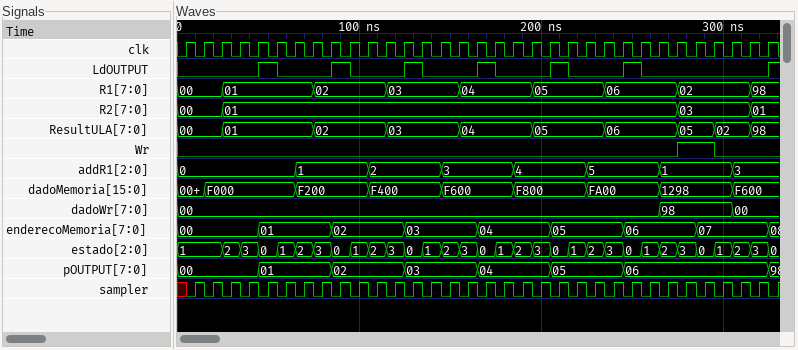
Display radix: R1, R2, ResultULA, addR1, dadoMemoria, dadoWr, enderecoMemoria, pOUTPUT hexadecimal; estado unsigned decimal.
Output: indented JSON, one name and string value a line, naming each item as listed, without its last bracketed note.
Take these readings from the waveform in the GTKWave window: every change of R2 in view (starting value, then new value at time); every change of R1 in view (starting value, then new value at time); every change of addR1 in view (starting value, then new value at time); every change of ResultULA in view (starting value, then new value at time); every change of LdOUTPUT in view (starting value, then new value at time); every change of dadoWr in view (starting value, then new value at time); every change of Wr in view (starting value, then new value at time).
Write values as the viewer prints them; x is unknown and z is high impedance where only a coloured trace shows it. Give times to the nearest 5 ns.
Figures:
{
  "every change of R2 in view": "00, 01 at 25 ns, 03 at 275 ns, 01 at 315 ns",
  "every change of R1 in view": "00, 01 at 25 ns, 02 at 75 ns, 03 at 115 ns, 04 at 155 ns, 05 at 195 ns, 06 at 235 ns, 02 at 275 ns, 98 at 315 ns",
  "every change of addR1 in view": "0, 1 at 65 ns, 2 at 105 ns, 3 at 145 ns, 4 at 185 ns, 5 at 225 ns, 1 at 265 ns, 3 at 305 ns",
  "every change of ResultULA in view": "00, 01 at 25 ns, 02 at 75 ns, 03 at 115 ns, 04 at 155 ns, 05 at 195 ns, 06 at 235 ns, 05 at 275 ns, 02 at 295 ns, 98 at 315 ns",
  "every change of LdOUTPUT in view": "0, 1 at 45 ns, 0 at 55 ns, 1 at 85 ns, 0 at 95 ns, 1 at 125 ns, 0 at 135 ns, 1 at 165 ns, 0 at 175 ns, 1 at 205 ns, 0 at 215 ns, 1 at 245 ns, 0 at 255 ns, 1 at 325 ns",
  "every change of dadoWr in view": "00, 98 at 265 ns, 00 at 305 ns",
  "every change of Wr in view": "0, 1 at 275 ns, 0 at 295 ns"
}
